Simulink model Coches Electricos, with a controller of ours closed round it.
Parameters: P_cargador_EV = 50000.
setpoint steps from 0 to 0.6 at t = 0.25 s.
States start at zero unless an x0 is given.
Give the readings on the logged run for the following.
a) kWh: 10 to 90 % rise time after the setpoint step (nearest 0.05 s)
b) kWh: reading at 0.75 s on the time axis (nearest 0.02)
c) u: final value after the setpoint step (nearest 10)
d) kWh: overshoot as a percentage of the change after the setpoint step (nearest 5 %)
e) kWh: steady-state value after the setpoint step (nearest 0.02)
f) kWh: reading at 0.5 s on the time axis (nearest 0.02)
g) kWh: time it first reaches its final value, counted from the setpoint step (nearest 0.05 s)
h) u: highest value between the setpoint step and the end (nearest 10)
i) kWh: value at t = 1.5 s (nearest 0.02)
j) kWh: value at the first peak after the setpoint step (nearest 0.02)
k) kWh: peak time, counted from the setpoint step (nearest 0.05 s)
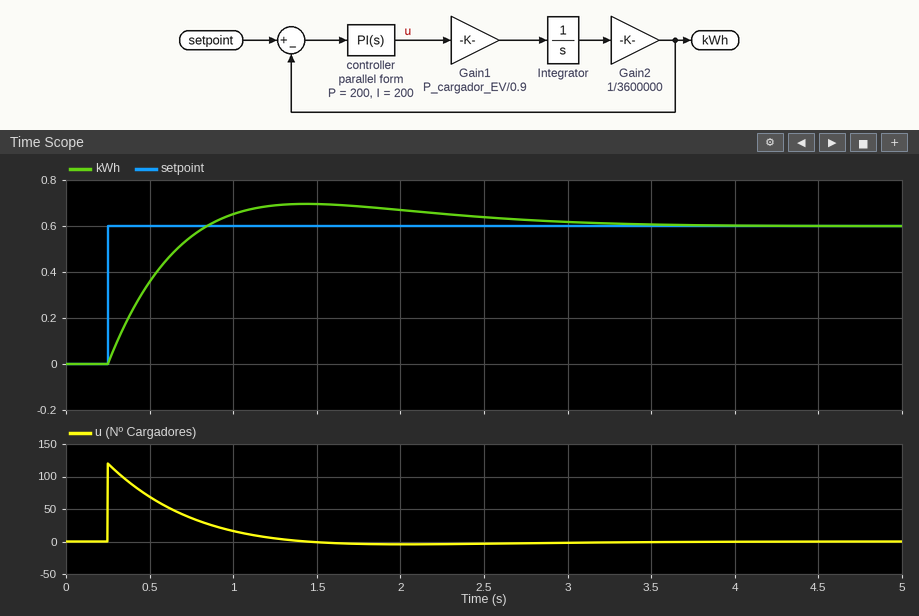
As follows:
0.45 s
0.56
0
15 %
0.60
0.36
0.60 s
120
0.70
0.70
1.20 s
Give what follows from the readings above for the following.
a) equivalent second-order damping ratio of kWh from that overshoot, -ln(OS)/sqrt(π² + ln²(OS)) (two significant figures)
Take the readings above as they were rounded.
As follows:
0.52
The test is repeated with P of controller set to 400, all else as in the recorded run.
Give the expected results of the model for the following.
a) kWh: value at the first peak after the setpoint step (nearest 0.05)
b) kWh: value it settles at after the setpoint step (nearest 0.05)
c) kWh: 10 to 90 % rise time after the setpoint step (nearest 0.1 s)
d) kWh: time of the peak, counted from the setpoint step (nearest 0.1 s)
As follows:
0.65
0.60
0.3 s
0.9 s
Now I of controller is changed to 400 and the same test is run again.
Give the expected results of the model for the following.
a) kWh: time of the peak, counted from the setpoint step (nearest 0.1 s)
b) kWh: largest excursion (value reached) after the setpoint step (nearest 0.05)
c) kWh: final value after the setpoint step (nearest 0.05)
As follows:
0.9 s
0.75
0.60
